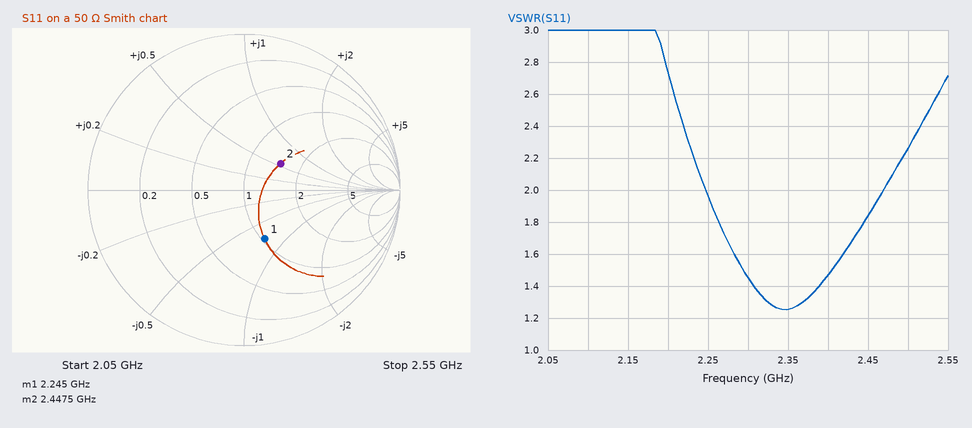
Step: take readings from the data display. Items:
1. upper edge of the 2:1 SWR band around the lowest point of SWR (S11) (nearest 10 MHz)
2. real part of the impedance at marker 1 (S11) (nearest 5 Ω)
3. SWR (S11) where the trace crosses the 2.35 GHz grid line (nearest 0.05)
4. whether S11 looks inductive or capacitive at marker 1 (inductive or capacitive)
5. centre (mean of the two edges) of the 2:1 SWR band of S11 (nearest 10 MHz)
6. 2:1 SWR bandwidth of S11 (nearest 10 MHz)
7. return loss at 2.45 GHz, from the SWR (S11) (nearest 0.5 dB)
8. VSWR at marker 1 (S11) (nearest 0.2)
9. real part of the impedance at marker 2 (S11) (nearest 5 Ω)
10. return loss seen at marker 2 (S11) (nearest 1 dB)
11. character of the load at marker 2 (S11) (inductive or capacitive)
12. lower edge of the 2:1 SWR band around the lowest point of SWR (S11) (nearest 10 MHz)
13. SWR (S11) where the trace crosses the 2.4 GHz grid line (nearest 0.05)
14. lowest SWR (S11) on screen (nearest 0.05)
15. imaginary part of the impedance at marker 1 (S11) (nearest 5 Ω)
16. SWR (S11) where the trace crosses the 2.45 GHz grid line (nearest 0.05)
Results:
2.47 GHz
50 Ω
1.25
capacitive
2.36 GHz
220 MHz
10.5 dB
2.0
75 Ω
11 dB
inductive
2.25 GHz
1.45
1.25
-35 Ω
1.85
